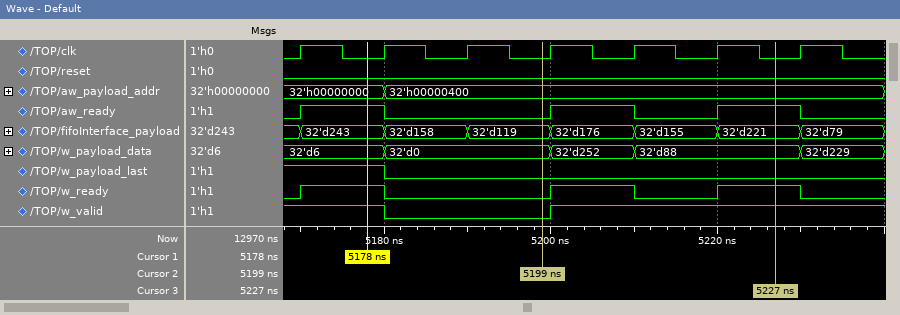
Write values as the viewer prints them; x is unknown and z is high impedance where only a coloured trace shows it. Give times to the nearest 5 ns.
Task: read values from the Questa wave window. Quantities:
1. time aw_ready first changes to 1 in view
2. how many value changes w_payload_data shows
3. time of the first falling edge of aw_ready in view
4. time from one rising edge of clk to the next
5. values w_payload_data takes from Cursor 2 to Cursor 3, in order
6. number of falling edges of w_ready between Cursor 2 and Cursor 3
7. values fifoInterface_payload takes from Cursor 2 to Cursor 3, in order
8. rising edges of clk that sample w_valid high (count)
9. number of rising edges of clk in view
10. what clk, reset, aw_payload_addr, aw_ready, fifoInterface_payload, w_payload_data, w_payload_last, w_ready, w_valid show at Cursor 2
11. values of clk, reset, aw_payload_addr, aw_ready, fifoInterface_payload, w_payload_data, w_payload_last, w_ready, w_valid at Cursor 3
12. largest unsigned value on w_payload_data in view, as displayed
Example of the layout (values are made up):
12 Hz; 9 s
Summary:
5170 ns; 4; 5180 ns; 10 ns; 32'd0, 32'd252, 32'd88; 1; 32'd119, 32'd176, 32'd155, 32'd221; 5; 7; clk=0, reset=0, aw_payload_addr=32'h00000400, aw_ready=0, fifoInterface_payload=32'd119, w_payload_data=32'd0, w_payload_last=0, w_ready=0, w_valid=0; clk=0, reset=0, aw_payload_addr=32'h00000400, aw_ready=1, fifoInterface_payload=32'd221, w_payload_data=32'd88, w_payload_last=0, w_ready=1, w_valid=1; 32'd252
